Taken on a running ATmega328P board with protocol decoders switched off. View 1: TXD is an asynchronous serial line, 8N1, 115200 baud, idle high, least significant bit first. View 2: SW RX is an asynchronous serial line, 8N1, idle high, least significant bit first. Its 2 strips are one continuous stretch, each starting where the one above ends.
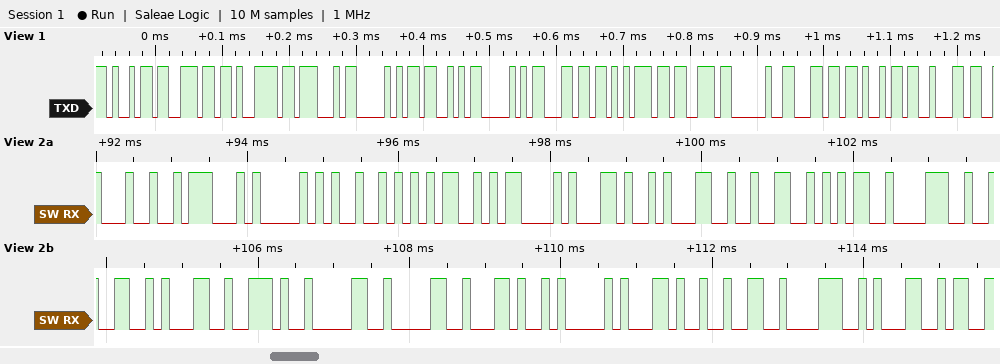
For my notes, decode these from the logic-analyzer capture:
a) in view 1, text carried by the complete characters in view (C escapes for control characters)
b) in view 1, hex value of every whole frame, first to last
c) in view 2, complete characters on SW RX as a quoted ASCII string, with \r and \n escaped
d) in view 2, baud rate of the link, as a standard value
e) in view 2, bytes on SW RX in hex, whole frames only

"inyGPSPlus lib"
69 6E 79 47 50 53 50 6C 75 73 20 6C 69 62
"$GPRMC,125821.00,A,281"
9600 baud
24 47 50 52 4D 43 2C 31 32 35 38 32 31 2E 30 30 2C 41 2C 32 38 31
